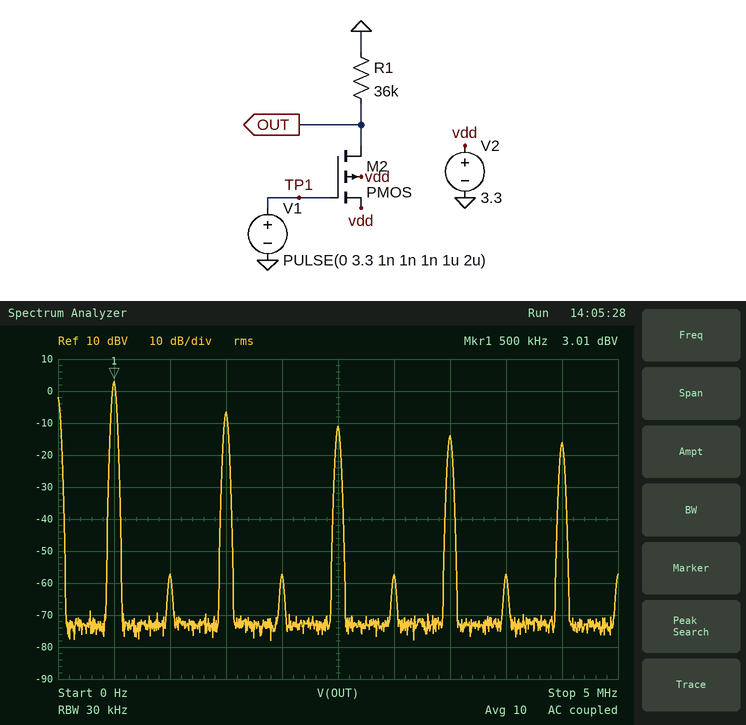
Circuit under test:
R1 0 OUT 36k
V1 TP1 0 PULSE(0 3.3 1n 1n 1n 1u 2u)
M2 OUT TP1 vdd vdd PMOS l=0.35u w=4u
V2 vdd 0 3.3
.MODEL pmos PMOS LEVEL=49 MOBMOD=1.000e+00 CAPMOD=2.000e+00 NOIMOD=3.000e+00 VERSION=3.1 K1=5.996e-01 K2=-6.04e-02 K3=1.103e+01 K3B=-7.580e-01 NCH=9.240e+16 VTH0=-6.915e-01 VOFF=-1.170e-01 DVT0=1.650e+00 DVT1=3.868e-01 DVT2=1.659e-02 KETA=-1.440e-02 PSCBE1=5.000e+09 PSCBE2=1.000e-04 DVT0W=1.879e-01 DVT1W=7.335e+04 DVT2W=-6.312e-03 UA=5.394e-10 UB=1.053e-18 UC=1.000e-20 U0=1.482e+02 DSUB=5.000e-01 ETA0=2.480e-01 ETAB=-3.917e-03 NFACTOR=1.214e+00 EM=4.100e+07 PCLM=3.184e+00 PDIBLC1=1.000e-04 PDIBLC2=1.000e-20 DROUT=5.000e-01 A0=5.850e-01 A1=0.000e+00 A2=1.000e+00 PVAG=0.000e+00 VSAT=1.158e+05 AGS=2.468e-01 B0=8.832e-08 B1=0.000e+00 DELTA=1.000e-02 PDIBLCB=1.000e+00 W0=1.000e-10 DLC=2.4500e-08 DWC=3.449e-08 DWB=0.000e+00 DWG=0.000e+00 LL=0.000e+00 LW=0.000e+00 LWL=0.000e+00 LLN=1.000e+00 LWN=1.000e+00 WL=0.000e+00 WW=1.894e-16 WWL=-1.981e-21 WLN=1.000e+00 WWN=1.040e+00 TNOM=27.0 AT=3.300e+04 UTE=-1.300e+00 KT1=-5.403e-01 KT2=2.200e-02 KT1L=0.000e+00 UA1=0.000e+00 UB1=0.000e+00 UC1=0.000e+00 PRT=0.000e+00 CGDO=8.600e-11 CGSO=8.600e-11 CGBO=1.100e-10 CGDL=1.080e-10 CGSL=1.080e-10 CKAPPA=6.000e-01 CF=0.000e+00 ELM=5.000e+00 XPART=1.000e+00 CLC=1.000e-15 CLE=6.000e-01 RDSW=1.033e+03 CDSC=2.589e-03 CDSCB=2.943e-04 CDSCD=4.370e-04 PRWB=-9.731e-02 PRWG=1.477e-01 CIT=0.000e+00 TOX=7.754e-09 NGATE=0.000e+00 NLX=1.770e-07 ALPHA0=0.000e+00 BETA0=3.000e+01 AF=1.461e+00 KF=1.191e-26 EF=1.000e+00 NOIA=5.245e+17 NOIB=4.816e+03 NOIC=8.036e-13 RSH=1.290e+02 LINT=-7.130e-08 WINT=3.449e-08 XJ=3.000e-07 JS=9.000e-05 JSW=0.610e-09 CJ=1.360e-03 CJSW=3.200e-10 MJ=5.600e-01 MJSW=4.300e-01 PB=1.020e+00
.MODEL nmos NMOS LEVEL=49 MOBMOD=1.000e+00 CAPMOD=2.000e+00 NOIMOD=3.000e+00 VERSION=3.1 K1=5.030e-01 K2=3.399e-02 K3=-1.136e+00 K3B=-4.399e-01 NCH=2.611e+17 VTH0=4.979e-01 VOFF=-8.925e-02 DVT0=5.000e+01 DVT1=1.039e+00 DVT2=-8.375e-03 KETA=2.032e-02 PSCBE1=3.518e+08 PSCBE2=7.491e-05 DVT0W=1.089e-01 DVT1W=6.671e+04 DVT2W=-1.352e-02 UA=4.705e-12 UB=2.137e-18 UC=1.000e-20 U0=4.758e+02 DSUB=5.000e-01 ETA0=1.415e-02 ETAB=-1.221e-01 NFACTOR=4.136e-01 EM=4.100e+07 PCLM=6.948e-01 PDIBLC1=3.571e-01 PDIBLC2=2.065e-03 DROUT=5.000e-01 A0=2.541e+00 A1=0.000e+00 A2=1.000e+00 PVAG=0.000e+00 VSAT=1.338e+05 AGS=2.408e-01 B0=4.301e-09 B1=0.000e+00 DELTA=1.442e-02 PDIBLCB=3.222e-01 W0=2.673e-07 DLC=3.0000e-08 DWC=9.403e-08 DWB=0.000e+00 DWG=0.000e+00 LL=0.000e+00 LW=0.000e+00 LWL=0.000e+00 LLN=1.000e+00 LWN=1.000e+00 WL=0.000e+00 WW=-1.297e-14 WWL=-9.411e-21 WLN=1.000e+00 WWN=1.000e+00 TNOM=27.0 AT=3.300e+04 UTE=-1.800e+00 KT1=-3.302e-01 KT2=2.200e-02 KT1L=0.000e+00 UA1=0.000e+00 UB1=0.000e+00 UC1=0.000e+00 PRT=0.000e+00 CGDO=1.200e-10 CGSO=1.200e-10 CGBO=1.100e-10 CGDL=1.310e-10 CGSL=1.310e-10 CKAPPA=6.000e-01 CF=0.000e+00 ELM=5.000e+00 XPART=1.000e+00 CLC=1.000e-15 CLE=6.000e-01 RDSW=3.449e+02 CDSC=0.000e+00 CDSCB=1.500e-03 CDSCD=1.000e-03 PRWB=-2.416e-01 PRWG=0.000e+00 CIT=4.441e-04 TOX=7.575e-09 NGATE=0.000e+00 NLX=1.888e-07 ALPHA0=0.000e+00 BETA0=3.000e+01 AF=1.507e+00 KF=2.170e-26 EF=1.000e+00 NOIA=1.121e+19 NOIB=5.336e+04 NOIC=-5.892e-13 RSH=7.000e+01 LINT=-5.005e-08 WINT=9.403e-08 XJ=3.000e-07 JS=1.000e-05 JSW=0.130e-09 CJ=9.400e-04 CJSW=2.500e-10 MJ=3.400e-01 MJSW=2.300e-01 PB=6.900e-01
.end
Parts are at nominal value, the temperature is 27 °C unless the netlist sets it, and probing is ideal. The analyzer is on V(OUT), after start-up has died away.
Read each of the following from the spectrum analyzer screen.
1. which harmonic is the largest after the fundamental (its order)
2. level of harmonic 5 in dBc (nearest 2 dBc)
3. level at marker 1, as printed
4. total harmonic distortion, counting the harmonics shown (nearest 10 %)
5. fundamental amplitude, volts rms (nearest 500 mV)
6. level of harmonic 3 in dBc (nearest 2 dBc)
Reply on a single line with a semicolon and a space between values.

3; -14 dBc; 3.01 dBV; 40 %; 1.5 V; -10 dBc
